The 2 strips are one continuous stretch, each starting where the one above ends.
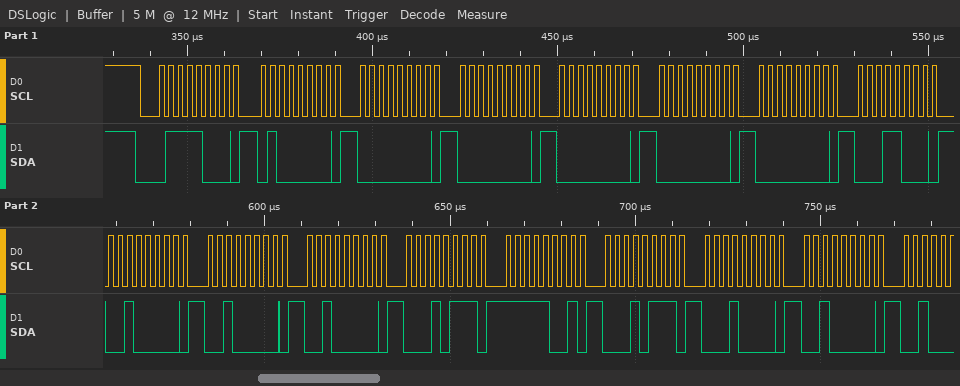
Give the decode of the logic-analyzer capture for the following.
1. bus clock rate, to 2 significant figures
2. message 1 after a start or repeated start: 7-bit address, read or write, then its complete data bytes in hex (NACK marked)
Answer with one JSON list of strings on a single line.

["400 kHz", "0x3C write: 40 00 00 00 00 00 18 20 20 20 17 F9 17 10 20"]
